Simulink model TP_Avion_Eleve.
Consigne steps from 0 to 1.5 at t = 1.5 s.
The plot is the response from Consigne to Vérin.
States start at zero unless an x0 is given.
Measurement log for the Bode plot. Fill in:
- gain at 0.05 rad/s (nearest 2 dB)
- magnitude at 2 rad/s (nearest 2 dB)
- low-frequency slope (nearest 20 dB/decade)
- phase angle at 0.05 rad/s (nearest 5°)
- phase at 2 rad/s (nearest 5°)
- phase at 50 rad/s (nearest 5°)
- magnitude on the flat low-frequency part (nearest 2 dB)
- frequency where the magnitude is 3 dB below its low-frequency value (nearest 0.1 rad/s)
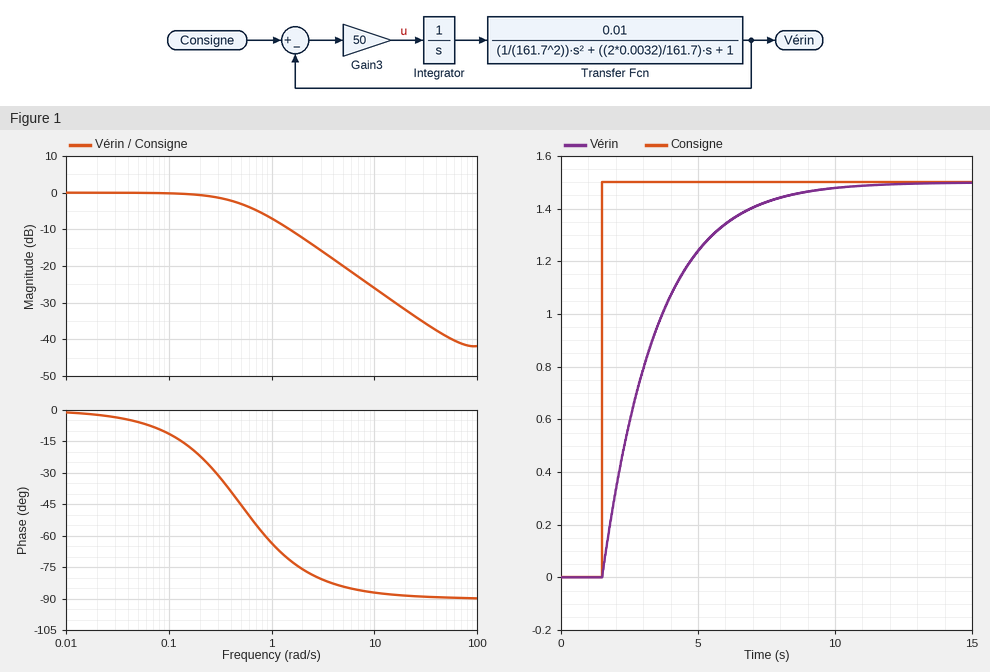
0 dB
-12 dB
0 dB/decade
-5°
-75°
-90°
0 dB
0.5 rad/s
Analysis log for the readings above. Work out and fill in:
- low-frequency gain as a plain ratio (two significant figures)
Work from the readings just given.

1.0
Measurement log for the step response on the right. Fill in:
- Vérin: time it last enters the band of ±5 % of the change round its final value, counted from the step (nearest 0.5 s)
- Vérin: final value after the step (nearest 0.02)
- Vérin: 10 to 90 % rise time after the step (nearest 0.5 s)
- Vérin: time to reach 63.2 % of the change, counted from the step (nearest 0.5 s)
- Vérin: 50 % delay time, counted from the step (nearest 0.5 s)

6.0 s
1.50
4.5 s
2.0 s
1.5 s
